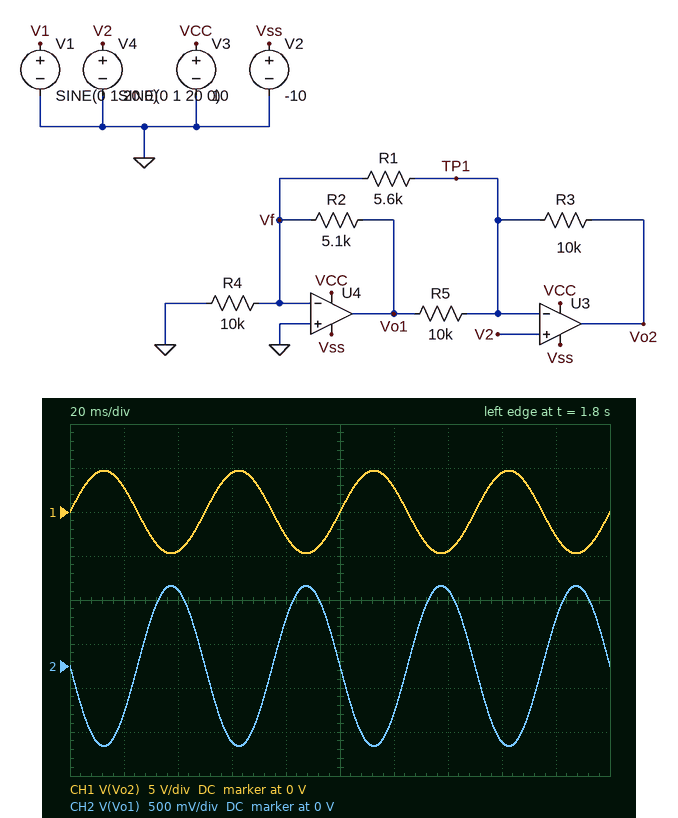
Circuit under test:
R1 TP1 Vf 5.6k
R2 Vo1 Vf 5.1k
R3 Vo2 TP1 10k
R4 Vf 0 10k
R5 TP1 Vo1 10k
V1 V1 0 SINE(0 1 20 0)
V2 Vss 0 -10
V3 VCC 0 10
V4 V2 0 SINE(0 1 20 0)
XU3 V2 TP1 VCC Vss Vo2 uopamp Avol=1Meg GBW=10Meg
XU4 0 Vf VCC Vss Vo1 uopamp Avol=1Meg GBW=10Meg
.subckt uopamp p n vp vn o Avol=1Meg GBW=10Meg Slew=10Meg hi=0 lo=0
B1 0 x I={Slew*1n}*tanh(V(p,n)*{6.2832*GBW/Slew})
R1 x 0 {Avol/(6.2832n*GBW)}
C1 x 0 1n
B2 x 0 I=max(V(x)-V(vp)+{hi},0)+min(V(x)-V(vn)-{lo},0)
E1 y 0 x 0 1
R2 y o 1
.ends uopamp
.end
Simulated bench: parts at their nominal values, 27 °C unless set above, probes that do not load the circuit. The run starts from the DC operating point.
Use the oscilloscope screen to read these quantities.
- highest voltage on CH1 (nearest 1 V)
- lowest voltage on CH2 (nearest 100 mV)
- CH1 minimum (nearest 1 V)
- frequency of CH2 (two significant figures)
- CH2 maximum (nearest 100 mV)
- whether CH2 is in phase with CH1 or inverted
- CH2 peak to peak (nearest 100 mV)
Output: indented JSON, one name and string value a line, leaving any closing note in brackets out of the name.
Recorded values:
{
  "highest voltage on CH1": "5 V",
  "lowest voltage on CH2": "-900 mV",
  "CH1 minimum": "-5 V",
  "frequency of CH2": "20 Hz",
  "CH2 maximum": "900 mV",
  "whether CH2 is in phase with CH1 or inverted": "inverted",
  "CH2 peak to peak": "1.8 V"
}
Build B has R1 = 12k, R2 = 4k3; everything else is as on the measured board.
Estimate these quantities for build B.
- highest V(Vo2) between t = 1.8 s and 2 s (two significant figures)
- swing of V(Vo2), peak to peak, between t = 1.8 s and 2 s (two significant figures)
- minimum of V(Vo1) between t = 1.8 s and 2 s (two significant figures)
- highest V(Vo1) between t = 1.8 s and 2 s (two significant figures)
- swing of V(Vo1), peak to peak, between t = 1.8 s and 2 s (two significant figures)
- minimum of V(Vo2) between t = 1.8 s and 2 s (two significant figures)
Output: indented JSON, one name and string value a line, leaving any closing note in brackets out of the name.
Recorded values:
{
  "highest V(Vo2) between t = 1.8 s and 2 s": "3.2 V",
  "swing of V(Vo2), peak to peak, between t = 1.8 s and 2 s": "6.4 V",
  "minimum of V(Vo1) between t = 1.8 s and 2 s": "-360 mV",
  "highest V(Vo1) between t = 1.8 s and 2 s": "360 mV",
  "swing of V(Vo1), peak to peak, between t = 1.8 s and 2 s": "720 mV",
  "minimum of V(Vo2) between t = 1.8 s and 2 s": "-3.2 V"
}
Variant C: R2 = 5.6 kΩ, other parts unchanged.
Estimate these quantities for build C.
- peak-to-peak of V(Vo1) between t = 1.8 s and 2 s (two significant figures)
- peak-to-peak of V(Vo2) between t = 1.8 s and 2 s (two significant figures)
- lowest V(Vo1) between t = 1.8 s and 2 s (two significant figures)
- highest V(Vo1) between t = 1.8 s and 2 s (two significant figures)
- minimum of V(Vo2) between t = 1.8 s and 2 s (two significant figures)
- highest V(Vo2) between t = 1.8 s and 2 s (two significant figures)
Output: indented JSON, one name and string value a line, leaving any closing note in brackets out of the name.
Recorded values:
{
  "peak-to-peak of V(Vo1) between t = 1.8 s and 2 s": "2.0 V",
  "peak-to-peak of V(Vo2) between t = 1.8 s and 2 s": "9.6 V",
  "lowest V(Vo1) between t = 1.8 s and 2 s": "-1.0 V",
  "highest V(Vo1) between t = 1.8 s and 2 s": "1.0 V",
  "minimum of V(Vo2) between t = 1.8 s and 2 s": "-4.8 V",
  "highest V(Vo2) between t = 1.8 s and 2 s": "4.8 V"
}
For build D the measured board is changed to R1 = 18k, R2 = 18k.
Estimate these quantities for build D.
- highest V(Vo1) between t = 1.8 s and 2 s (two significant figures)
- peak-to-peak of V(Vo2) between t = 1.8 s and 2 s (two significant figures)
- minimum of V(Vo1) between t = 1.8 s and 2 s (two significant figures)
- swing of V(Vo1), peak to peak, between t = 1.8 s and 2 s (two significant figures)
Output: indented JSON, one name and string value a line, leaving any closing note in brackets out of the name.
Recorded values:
{
  "highest V(Vo1) between t = 1.8 s and 2 s": "1.0 V",
  "peak-to-peak of V(Vo2) between t = 1.8 s and 2 s": "7.1 V",
  "minimum of V(Vo1) between t = 1.8 s and 2 s": "-1.0 V",
  "swing of V(Vo1), peak to peak, between t = 1.8 s and 2 s": "2.0 V"
}
